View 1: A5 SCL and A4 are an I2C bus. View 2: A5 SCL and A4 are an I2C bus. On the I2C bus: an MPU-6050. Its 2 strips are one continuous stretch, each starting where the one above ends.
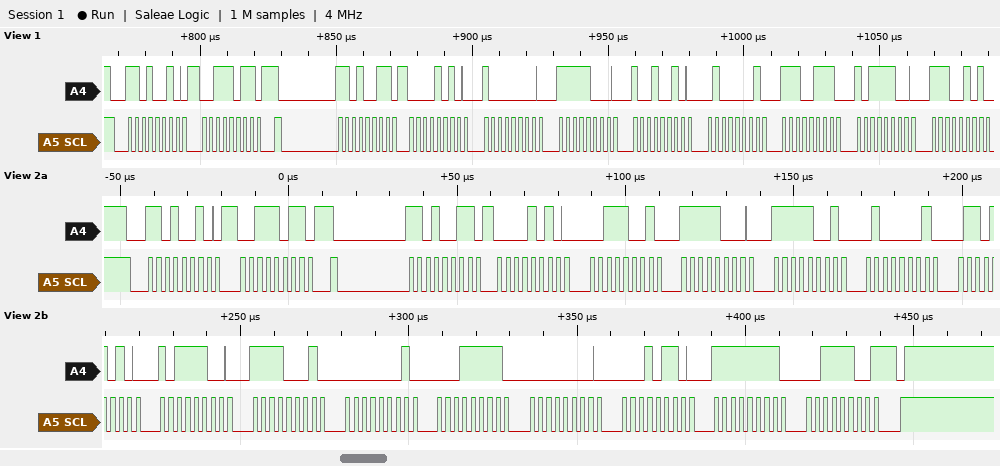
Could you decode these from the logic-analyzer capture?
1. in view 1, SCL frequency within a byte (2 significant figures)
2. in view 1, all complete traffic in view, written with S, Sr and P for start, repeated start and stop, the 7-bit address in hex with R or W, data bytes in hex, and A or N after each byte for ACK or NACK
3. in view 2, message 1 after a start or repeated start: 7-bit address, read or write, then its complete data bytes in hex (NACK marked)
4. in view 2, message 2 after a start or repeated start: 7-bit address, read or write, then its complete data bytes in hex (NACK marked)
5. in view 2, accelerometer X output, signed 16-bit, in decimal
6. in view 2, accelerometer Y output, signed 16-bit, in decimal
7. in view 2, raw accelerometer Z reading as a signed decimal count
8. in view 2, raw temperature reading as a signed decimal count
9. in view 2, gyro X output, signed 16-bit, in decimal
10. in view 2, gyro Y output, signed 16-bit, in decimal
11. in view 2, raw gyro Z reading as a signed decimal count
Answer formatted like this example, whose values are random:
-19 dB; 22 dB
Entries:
400 kHz; S 69W A 3B A Sr 69R A 0A A 80 A F8 A 92 A 41 A E7 A BC A E5 A; 0x69 write: 3B; 0x69 read: 0A 39 F8 F9 41 6A BC F1 01 1F 00 16 FF 3C NACK; 2617; -1799; 16746; -17167; 287; 22; -196
